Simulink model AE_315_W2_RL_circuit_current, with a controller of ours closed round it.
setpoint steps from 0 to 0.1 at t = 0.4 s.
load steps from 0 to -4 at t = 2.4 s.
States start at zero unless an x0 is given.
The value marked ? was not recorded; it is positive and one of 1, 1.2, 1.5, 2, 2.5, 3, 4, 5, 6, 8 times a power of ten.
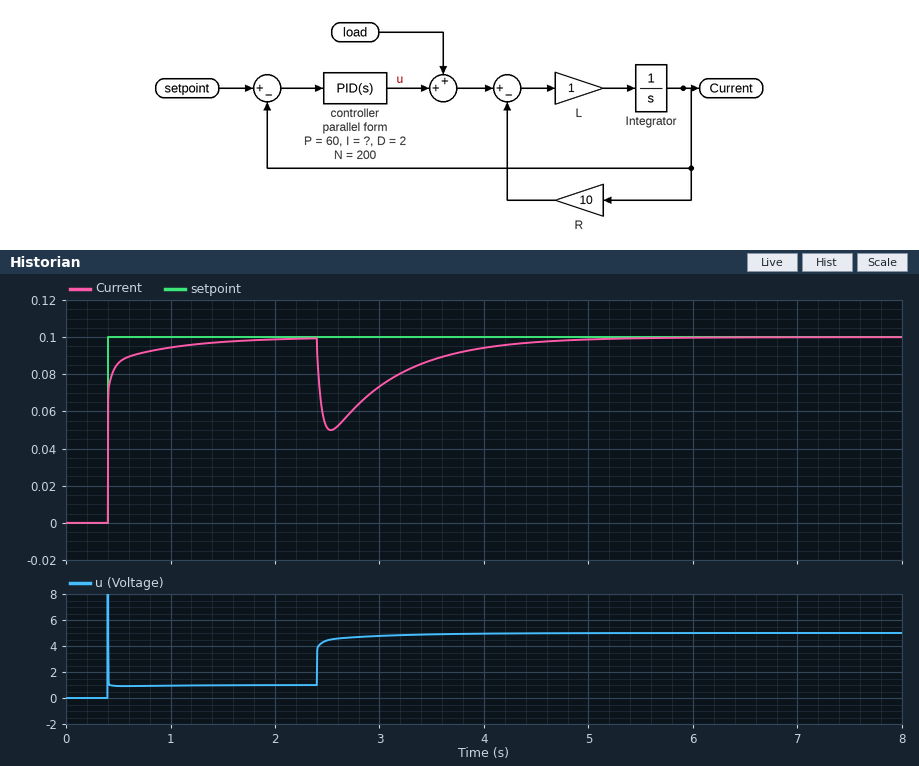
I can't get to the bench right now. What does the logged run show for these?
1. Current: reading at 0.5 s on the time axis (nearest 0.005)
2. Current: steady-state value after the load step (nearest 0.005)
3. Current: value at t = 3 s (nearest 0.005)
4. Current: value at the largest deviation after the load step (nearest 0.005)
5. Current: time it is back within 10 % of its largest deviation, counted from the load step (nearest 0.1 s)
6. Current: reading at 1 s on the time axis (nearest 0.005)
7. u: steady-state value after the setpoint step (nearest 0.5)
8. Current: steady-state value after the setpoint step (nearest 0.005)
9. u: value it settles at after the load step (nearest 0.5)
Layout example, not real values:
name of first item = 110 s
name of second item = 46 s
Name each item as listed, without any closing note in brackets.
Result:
Current: reading at 0.5 s on the time axis = 0.085
Current: steady-state value after the load step = 0.100
Current: value at t = 3 s = 0.075
Current: value at the largest deviation after the load step = 0.050
Current: time it is back within 10 % of its largest deviation, counted from the load step = 1.7 s
Current: reading at 1 s on the time axis = 0.095
u: steady-state value after the setpoint step = 1.0
Current: steady-state value after the setpoint step = 0.100
u: value it settles at after the load step = 5.0
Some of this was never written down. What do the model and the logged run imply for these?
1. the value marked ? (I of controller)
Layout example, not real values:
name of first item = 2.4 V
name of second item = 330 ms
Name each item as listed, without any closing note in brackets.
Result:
the value marked ? = 100
